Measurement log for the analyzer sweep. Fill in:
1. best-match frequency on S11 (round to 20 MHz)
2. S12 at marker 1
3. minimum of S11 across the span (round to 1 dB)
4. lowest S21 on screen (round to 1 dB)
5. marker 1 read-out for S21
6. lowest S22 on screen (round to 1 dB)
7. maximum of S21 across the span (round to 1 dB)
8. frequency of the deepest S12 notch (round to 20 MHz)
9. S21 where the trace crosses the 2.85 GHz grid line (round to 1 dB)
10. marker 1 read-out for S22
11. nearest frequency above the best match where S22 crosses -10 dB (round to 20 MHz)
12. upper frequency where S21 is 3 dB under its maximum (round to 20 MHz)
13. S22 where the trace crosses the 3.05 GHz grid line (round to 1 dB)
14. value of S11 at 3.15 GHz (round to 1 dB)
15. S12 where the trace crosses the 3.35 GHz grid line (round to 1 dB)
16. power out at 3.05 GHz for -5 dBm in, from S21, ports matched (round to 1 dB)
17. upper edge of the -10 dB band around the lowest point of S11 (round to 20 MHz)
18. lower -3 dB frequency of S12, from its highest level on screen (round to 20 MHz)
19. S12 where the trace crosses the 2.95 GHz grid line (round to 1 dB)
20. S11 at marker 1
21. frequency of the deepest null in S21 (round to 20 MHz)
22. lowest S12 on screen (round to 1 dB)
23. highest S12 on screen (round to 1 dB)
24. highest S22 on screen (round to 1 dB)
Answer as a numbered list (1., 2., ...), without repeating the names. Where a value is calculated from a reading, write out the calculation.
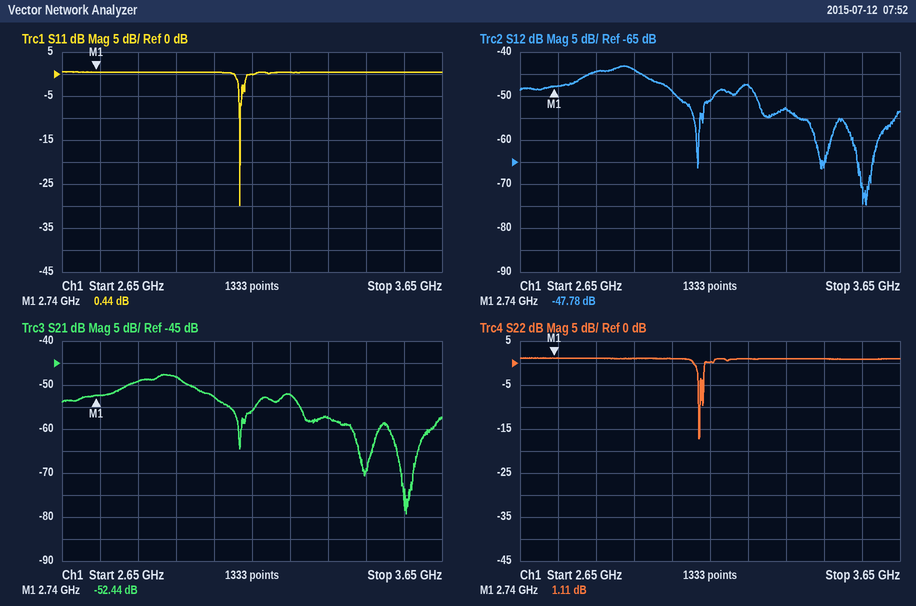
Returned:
1. 3.12 GHz
2. -47.78 dB
3. -30 dB
4. -79 dB
5. -52.44 dB
6. -17 dB
7. -48 dB
8. 3.56 GHz
9. -49 dB
10. 1.11 dB
11. 3.12 GHz
12. 3.00 GHz
13. 1 dB
14. 0 dB
15. -53 dB
16. -5 dBm + (-53 dB) = -58 dBm
17. 3.12 GHz
18. 2.80 GHz
19. -44 dB
20. 0.44 dB
21. 3.56 GHz
22. -75 dB
23. -43 dB
24. 1 dB
